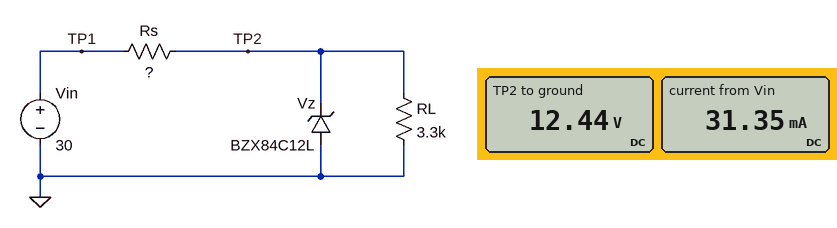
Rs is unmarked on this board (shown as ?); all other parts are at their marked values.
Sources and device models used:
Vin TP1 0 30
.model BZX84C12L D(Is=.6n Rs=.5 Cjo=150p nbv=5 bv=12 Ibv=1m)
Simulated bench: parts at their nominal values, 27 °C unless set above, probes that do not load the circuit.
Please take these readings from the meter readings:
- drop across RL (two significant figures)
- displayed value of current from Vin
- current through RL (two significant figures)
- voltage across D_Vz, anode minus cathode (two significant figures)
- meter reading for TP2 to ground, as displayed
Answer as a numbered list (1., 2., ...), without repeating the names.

1. 12 V
2. 31.35 mA
3. 3.8 mA
4. -12 V
5. 12.44 V
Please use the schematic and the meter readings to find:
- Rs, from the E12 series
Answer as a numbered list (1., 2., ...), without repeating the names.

1. 560 Ω
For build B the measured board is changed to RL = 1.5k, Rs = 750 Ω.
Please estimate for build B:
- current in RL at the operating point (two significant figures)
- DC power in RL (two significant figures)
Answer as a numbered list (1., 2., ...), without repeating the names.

1. 8.2 mA
2. 100 mW
